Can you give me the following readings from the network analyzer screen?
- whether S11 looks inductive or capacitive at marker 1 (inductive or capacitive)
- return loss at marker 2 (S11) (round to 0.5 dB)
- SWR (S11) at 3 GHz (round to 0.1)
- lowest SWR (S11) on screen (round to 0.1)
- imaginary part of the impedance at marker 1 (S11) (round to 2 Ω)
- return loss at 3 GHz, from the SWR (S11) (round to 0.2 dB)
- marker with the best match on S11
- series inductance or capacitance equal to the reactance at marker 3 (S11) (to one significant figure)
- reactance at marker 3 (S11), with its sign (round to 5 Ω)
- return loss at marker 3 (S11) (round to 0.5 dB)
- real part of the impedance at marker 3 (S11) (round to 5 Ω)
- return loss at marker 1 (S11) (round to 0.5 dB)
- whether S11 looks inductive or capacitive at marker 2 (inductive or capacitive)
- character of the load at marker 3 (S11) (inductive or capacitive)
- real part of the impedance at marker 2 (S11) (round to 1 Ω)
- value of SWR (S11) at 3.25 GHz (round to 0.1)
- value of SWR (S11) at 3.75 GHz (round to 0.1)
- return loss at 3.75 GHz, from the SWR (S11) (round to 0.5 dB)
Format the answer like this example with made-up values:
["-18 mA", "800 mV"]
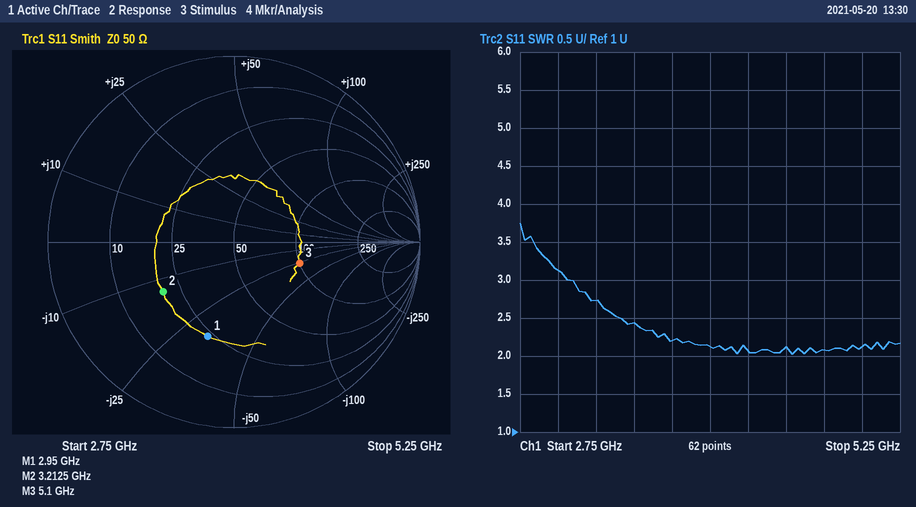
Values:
["capacitive", "6.5 dB", "3.1", "2.0", "-32 Ω", "5.8 dB", "marker 3", "1 pF", "-25 Ω", "8.5 dB", "100 Ω", "5.5 dB", "capacitive", "capacitive", "20 Ω", "2.7", "2.2", "8.5 dB"]
